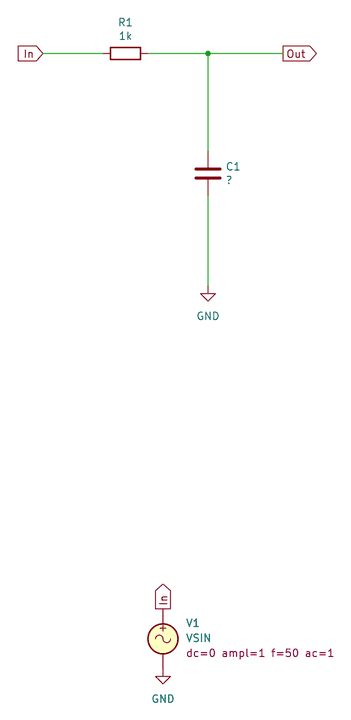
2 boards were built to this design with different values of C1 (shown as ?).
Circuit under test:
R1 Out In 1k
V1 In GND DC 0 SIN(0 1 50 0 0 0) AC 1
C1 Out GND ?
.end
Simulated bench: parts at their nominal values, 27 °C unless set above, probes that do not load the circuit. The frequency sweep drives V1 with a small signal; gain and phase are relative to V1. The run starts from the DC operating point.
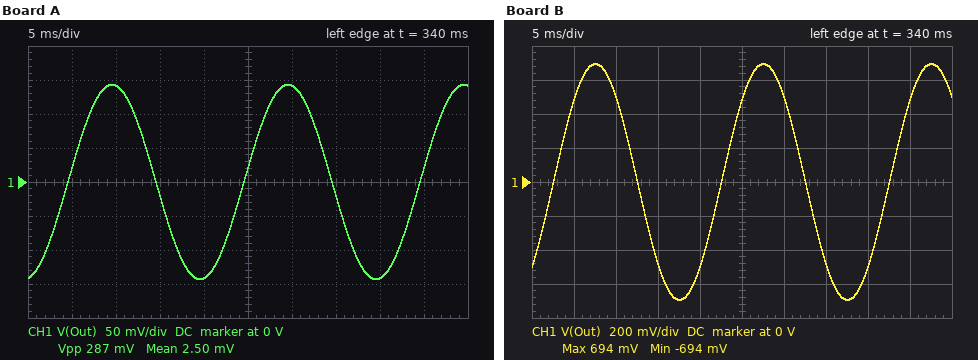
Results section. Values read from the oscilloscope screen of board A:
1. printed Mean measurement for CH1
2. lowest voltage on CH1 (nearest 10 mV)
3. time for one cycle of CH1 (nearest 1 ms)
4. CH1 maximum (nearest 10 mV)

2.50 mV
-140 mV
20 ms
140 mV
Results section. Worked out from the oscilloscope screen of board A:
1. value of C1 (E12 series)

22 µF
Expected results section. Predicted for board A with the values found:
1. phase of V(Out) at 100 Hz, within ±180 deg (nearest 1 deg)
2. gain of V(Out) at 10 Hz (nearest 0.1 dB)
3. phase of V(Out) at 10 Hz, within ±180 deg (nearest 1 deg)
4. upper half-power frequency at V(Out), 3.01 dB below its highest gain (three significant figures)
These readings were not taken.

-86 deg
-4.6 dB
-54 deg
7.23 Hz
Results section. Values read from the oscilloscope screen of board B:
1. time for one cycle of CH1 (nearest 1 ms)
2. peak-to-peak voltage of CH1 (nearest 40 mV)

20 ms
1.40 V
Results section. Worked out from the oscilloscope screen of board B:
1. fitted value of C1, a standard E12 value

3.3 µF
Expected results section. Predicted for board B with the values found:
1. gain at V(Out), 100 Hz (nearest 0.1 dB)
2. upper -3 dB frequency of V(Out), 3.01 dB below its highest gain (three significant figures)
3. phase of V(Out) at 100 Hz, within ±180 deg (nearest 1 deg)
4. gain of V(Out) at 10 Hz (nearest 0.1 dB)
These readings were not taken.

-7.2 dB
48.2 Hz
-64 deg
-0.2 dB
